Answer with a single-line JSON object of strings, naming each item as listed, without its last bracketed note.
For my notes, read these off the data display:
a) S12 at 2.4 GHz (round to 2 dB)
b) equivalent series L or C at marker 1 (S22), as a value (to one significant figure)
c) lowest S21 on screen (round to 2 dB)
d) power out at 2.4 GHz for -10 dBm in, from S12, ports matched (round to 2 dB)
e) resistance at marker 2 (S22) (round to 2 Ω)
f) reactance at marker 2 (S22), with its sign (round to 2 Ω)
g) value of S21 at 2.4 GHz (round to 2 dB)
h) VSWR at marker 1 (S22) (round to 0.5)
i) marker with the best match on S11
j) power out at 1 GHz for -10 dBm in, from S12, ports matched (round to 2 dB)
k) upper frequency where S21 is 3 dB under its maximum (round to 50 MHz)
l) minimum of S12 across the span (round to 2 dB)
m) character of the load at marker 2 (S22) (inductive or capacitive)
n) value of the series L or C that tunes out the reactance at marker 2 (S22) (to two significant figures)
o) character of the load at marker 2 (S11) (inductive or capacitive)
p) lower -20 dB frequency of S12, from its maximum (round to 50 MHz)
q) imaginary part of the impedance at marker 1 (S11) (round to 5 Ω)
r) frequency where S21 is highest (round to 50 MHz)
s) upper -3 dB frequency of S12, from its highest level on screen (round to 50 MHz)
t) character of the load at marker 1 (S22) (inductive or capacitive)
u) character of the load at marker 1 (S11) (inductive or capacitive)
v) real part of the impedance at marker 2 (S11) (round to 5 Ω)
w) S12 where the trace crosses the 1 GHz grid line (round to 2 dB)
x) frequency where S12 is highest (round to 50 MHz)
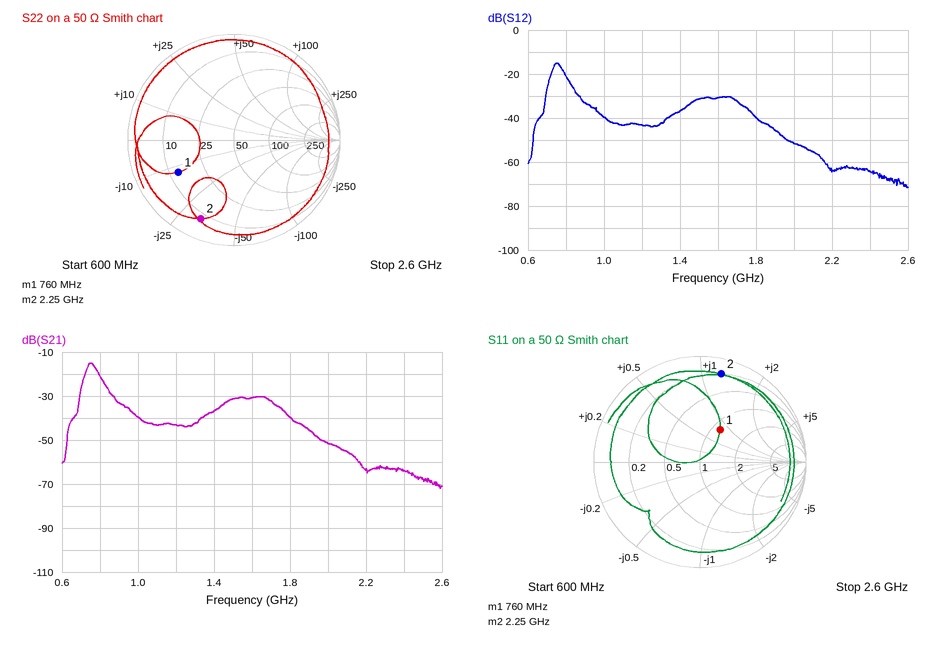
{"S12 at 2.4 GHz": "-64 dB", "equivalent series L or C at marker 1 (S22), as a value": "20 pF", "lowest S21 on screen": "-72 dB", "power out at 2.4 GHz for -10 dBm in, from S12, ports matched": "-74 dBm", "resistance at marker 2 (S22)": "8 Ω", "reactance at marker 2 (S22), with its sign": "-32 Ω", "value of S21 at 2.4 GHz": "-64 dB", "VSWR at marker 1 (S22)": "4.0", "marker with the best match on S11": "marker 1", "power out at 1 GHz for -10 dBm in, from S12, ports matched": "-50 dBm", "upper frequency where S21 is 3 dB under its maximum": "800 MHz", "minimum of S12 across the span": "-72 dB", "character of the load at marker 2 (S22)": "capacitive", "value of the series L or C that tunes out the reactance at marker 2 (S22)": "2.3 nH", "character of the load at marker 2 (S11)": "inductive", "lower -20 dB frequency of S12, from its maximum": "700 MHz", "imaginary part of the impedance at marker 1 (S11)": "+40 Ω", "frequency where S21 is highest": "750 MHz", "upper -3 dB frequency of S12, from its highest level on screen": "800 MHz", "character of the load at marker 1 (S22)": "capacitive", "character of the load at marker 1 (S11)": "inductive", "real part of the impedance at marker 2 (S11)": "10 Ω", "S12 where the trace crosses the 1 GHz grid line": "-40 dB", "frequency where S12 is highest": "750 MHz"}
